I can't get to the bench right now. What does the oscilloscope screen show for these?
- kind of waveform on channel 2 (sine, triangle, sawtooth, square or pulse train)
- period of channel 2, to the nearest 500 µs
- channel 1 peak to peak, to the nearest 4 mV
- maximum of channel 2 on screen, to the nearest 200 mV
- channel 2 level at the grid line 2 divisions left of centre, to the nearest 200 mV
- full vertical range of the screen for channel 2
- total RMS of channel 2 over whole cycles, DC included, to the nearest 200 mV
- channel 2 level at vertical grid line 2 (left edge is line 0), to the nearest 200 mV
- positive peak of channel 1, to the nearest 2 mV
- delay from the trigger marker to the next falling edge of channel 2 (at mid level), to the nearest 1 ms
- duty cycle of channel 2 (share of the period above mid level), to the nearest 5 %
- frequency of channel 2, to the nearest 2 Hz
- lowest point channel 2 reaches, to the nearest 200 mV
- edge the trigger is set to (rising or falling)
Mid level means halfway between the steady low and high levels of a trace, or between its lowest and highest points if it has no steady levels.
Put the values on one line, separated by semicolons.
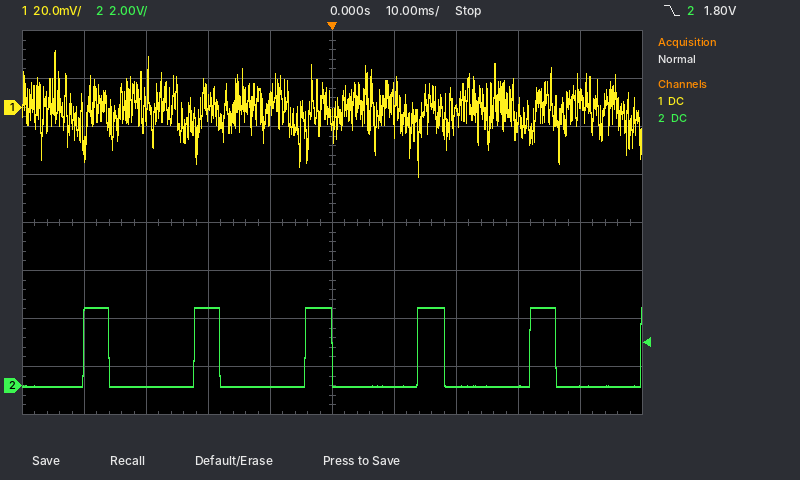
pulse train; 18.0 ms; 52 mV; 3.2 V; 3.2 V; 16 V; 1.6 V; 0.0 V; 24 mV; 18 ms; 25 %; 56 Hz; 0.0 V; falling
